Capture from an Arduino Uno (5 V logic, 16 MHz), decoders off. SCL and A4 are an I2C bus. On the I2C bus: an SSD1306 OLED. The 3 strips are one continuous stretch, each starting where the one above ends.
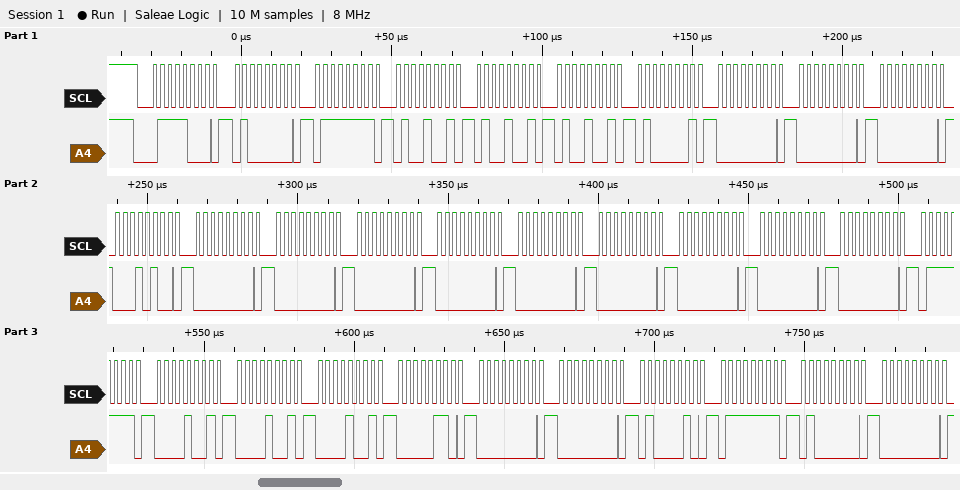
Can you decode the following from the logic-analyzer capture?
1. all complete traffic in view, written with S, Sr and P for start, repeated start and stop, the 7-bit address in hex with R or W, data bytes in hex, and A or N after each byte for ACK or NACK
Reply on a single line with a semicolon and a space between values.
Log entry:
S 3CW A 40 A 7F A 49 A 49 A 49 A 41 A 00 A 00 A 00 A 14 A 00 A 00 A 00 A 00 A 00 A 00 A 00 A 00 A 00 A 7F A 09 A 09 A 09 A 06 A 00 A 00 A 42 A 7F A 40 A 00 A
